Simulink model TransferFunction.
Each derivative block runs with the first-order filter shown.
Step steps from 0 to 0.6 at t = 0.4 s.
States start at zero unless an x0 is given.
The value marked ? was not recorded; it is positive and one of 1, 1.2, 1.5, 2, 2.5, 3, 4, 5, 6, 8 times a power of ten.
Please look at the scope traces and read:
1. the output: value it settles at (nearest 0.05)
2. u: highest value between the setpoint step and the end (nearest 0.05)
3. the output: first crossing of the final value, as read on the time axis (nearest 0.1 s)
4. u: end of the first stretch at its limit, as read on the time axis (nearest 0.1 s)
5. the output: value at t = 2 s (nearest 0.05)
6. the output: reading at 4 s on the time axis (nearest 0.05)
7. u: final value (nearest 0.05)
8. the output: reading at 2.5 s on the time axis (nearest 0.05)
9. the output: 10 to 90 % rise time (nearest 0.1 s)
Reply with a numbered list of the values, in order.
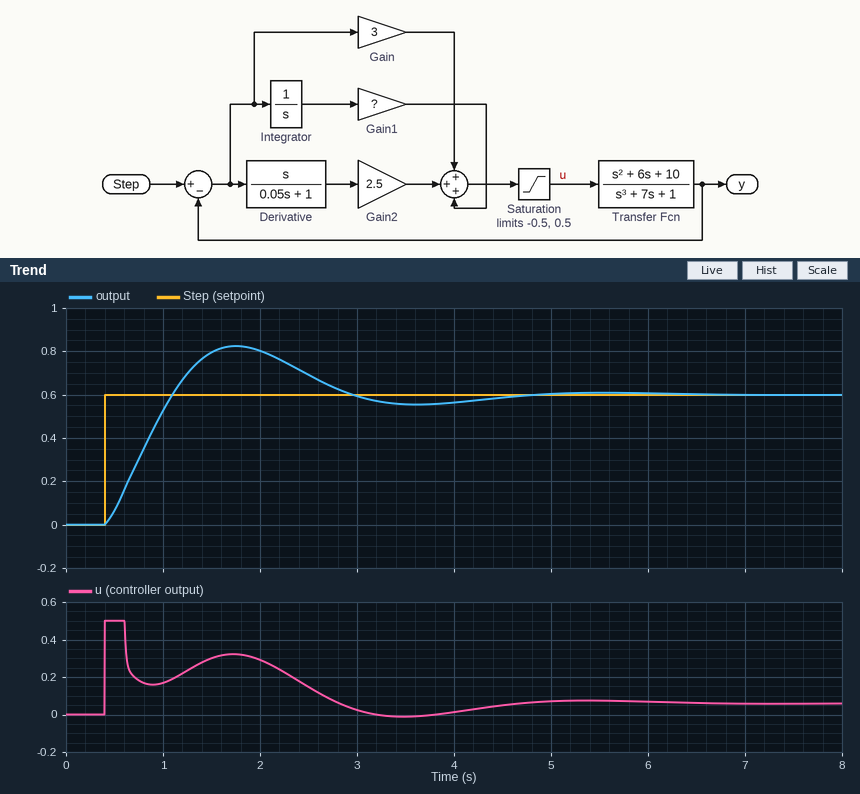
1. 0.60
2. 0.50
3. 1.1 s
4. 0.6 s
5. 0.80
6. 0.55
7. 0.05
8. 0.70
9. 0.5 s
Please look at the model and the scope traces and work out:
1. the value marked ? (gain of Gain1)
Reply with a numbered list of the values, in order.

1. 10
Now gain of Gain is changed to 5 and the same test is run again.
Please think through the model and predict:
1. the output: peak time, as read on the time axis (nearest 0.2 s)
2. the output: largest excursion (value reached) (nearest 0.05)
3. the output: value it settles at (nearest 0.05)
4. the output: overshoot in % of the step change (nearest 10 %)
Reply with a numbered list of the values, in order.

1. 1.6 s
2. 0.75
3. 0.60
4. 30 %
